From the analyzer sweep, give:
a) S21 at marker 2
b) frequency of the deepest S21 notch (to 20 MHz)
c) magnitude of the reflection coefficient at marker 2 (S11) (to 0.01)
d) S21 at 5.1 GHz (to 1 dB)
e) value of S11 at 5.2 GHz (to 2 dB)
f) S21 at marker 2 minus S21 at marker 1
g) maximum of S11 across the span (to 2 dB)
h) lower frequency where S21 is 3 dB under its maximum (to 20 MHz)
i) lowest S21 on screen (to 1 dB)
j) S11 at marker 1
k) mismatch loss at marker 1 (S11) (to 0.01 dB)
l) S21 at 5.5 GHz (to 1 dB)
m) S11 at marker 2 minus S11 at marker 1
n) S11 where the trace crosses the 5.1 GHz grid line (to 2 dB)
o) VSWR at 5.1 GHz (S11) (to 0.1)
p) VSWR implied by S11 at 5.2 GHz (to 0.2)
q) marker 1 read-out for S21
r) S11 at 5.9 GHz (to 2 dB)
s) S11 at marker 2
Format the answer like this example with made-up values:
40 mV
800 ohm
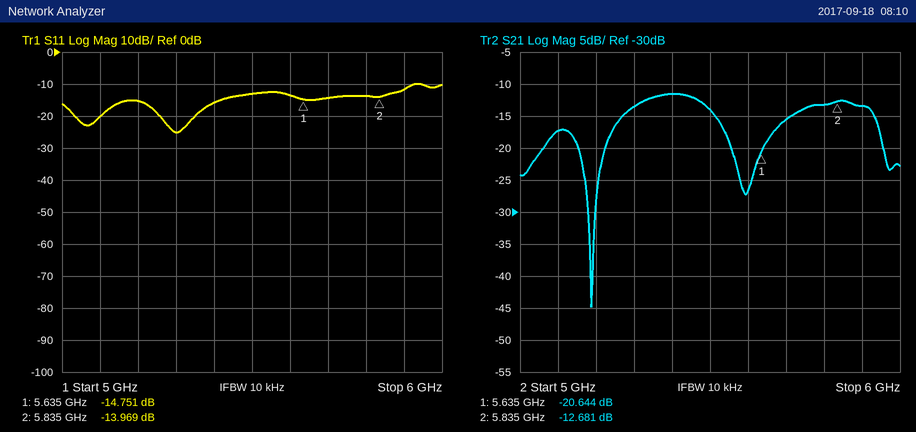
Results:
-12.681 dB
5.18 GHz
0.20
-17 dB
-16 dB
7.963 dB
-10 dB
5.28 GHz
-45 dB
-14.751 dB
0.15 dB
-14 dB
0.782 dB
-20 dB
1.2
1.4
-20.644 dB
-12 dB
-13.969 dB
